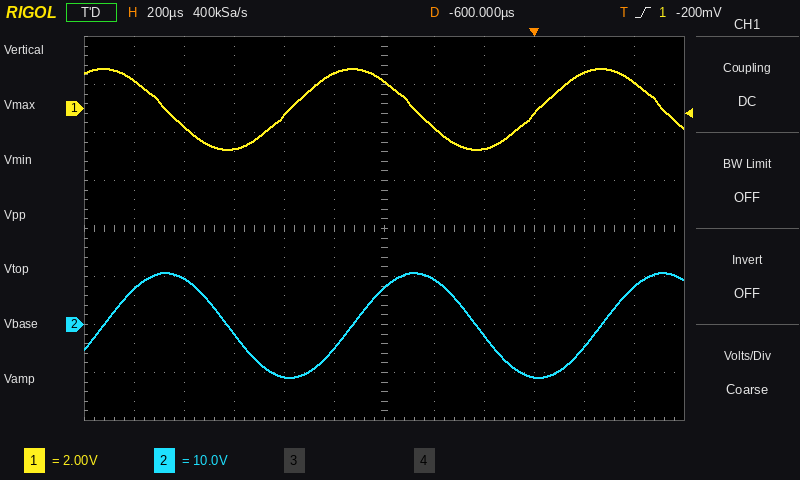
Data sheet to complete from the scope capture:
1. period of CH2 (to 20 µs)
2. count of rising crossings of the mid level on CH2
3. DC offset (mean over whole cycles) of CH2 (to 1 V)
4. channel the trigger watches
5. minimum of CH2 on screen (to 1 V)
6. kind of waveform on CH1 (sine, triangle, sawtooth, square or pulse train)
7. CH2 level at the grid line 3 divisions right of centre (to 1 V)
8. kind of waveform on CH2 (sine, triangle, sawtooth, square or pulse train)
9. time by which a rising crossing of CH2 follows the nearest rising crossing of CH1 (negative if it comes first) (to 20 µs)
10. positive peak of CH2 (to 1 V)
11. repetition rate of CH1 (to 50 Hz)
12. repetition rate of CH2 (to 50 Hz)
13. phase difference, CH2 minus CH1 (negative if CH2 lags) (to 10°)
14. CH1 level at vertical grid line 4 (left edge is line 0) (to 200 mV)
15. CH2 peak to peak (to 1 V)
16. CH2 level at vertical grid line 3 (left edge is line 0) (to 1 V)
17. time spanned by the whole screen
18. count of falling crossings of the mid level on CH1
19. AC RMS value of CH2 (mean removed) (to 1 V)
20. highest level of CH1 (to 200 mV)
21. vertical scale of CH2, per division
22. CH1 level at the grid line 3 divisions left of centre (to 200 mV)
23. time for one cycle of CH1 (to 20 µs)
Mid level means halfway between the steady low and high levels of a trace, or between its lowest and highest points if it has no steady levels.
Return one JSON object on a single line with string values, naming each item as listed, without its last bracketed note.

{"period of CH2": "1.00 ms", "count of rising crossings of the mid level on CH2": "3", "DC offset (mean over whole cycles) of CH2": "0 V", "channel the trigger watches": "CH1", "minimum of CH2 on screen": "-11 V", "kind of waveform on CH1": "sine", "CH2 level at the grid line 3 divisions right of centre": "-11 V", "kind of waveform on CH2": "sine", "time by which a rising crossing of CH2 follows the nearest rising crossing of CH1 (negative if it comes first)": "+260 µs", "positive peak of CH2": "11 V", "repetition rate of CH1": "1.00 kHz", "repetition rate of CH2": "1.00 kHz", "phase difference, CH2 minus CH1 (negative if CH2 lags)": "-90°", "CH1 level at vertical grid line 4 (left edge is line 0)": "-200 mV", "CH2 peak to peak": "22 V", "CH2 level at vertical grid line 3 (left edge is line 0)": "-2 V", "time spanned by the whole screen": "2.4 ms", "count of falling crossings of the mid level on CH1": "3", "AC RMS value of CH2 (mean removed)": "8 V", "highest level of CH1": "1.6 V", "vertical scale of CH2, per division": "10 V", "CH1 level at the grid line 3 divisions left of centre": "-1.6 V", "time for one cycle of CH1": "1.00 ms"}
